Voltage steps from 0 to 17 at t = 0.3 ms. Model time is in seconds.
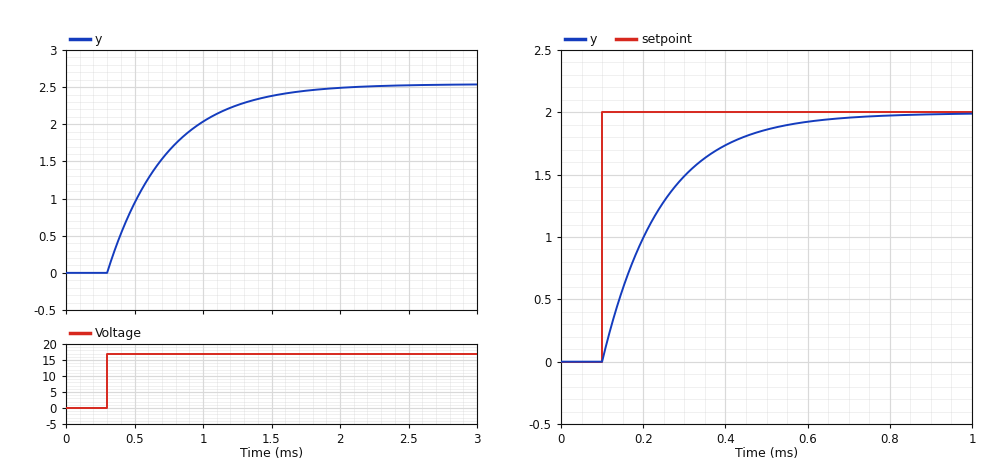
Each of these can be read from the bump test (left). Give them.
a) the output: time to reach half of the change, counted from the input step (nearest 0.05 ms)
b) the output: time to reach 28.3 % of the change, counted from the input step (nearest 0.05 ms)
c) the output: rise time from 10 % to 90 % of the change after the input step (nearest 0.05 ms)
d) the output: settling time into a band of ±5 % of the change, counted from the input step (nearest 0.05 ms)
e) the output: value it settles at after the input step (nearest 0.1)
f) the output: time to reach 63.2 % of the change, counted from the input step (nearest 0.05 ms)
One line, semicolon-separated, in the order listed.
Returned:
0.30 ms; 0.15 ms; 0.95 ms; 1.30 ms; 2.5; 0.45 ms
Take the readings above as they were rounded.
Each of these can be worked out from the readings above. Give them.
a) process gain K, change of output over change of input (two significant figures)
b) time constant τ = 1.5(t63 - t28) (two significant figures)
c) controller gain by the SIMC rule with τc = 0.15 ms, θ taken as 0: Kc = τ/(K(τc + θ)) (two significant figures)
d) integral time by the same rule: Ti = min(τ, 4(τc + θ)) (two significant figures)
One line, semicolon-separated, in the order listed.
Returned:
0.15; 0.45 ms; 20; 0.45 ms
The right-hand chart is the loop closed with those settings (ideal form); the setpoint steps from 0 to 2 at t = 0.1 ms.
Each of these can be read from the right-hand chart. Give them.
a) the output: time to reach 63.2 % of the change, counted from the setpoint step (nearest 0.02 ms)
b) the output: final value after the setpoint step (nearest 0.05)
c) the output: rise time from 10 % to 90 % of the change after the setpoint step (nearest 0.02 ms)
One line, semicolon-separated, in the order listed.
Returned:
0.14 ms; 2.00; 0.32 ms
